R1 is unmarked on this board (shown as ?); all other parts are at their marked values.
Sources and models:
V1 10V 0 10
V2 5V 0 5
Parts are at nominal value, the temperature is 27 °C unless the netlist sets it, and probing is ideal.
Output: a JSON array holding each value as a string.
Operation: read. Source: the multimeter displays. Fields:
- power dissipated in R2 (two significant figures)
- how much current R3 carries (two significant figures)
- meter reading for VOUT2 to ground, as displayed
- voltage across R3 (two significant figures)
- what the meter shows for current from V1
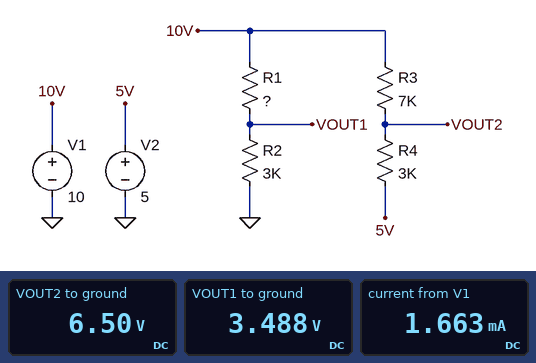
["4.1 mW", "500 µA", "6.50 V", "3.5 V", "1.663 mA"]
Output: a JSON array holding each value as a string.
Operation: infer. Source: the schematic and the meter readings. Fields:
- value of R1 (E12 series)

["5.6 kΩ"]
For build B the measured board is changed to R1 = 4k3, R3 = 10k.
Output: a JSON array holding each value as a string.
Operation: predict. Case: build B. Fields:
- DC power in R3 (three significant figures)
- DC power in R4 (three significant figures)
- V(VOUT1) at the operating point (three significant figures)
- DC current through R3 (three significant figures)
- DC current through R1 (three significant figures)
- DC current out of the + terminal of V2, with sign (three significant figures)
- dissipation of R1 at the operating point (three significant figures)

["1.48 mW", "444 µW", "4.11 V", "385 µA", "1.37 mA", "-385 µA", "8.07 mW"]
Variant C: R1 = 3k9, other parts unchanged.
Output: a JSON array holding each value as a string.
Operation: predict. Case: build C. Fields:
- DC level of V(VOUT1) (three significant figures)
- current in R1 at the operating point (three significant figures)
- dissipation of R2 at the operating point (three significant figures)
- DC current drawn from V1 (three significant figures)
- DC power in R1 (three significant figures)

["4.35 V", "1.45 mA", "6.30 mW", "1.95 mA", "8.19 mW"]
